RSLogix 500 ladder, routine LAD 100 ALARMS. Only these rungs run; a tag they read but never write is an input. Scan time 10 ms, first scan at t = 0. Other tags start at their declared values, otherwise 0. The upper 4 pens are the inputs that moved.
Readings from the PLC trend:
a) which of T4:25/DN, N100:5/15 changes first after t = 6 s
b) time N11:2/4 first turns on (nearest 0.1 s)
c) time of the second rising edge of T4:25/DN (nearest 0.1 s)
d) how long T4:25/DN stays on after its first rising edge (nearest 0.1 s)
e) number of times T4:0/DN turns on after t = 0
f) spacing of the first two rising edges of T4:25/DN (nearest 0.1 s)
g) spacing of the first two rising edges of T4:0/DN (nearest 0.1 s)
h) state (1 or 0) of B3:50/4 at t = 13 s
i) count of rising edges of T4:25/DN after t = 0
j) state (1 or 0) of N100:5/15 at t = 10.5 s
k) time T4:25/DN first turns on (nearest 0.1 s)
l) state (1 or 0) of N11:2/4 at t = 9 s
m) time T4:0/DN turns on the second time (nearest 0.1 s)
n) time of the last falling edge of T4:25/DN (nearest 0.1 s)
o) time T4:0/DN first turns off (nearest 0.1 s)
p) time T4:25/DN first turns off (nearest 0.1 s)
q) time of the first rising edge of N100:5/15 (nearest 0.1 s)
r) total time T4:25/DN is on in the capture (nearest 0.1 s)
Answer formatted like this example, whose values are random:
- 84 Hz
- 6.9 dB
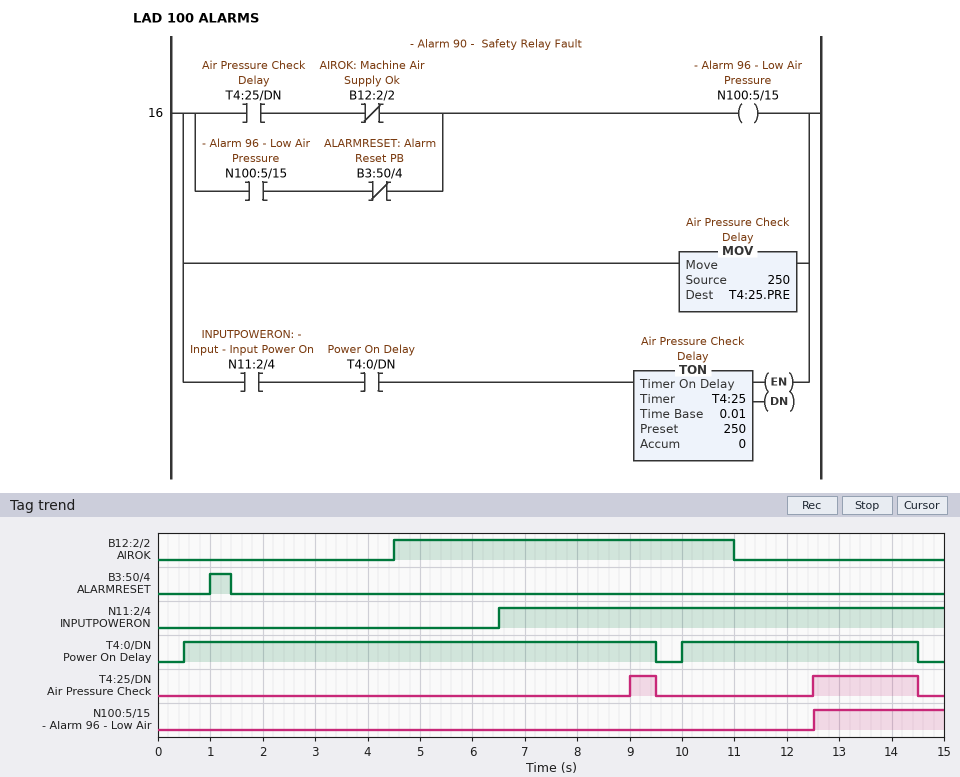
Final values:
- T4:25/DN
- 6.5 s
- 12.5 s
- 0.5 s
- 2
- 3.5 s
- 9.5 s
- 0
- 2
- 0
- 9.0 s
- 1
- 10.0 s
- 14.5 s
- 9.5 s
- 9.5 s
- 12.5 s
- 2.5 s
